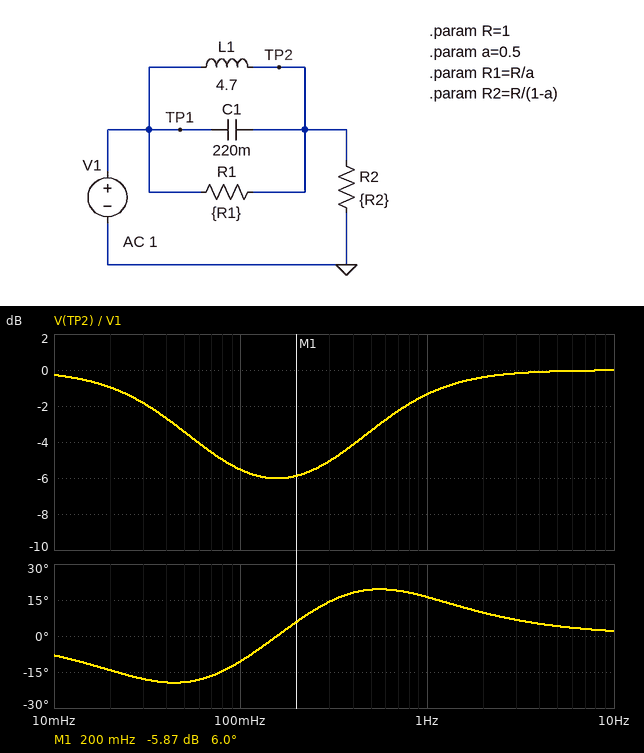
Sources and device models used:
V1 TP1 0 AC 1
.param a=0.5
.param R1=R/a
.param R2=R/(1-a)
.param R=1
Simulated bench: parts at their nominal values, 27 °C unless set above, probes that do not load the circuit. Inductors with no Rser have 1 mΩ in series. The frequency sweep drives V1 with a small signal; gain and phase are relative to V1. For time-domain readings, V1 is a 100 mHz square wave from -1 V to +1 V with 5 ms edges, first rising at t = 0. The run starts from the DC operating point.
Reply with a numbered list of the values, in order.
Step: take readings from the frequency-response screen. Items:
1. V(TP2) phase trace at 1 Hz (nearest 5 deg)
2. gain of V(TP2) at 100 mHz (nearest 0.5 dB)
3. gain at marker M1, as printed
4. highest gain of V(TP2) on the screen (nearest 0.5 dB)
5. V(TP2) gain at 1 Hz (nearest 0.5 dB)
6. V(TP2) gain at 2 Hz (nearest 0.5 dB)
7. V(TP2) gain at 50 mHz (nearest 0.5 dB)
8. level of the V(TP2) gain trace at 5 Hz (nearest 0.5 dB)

1. 15 deg
2. -5.5 dB
3. -5.87 dB
4. 0 dB
5. -1.5 dB
6. -0.5 dB
7. -3.5 dB
8. 0 dB
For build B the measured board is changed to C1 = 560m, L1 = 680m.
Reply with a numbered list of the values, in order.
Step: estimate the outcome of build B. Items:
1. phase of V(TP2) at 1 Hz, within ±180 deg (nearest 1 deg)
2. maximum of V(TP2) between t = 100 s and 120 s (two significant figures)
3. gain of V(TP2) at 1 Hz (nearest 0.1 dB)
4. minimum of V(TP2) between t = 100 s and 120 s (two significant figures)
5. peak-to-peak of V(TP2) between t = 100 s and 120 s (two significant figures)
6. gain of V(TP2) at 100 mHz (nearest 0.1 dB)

1. 8 deg
2. 1.1 V
3. -0.3 dB
4. -1.1 V
5. 2.1 V
6. -0.7 dB
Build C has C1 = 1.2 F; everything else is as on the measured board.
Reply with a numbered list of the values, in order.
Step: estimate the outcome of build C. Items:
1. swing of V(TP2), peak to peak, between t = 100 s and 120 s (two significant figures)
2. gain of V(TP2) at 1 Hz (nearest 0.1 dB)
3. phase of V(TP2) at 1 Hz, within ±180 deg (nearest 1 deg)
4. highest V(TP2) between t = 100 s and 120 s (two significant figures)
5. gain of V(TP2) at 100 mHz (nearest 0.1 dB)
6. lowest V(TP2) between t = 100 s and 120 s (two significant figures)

1. 2.8 V
2. -0.1 dB
3. 4 deg
4. 1.4 V
5. -4.4 dB
6. -1.4 V
